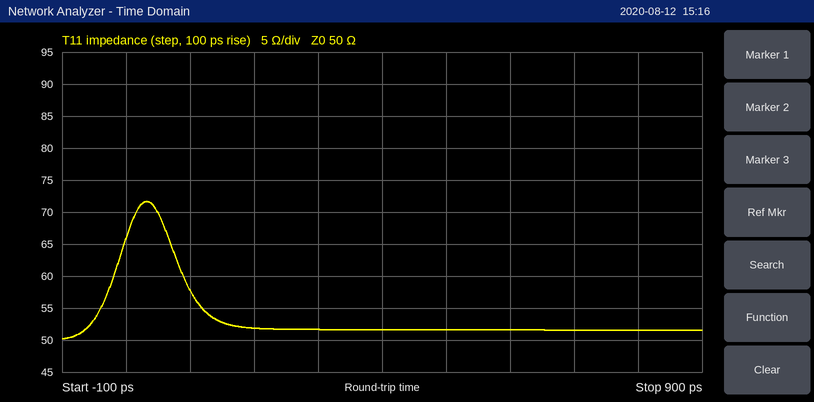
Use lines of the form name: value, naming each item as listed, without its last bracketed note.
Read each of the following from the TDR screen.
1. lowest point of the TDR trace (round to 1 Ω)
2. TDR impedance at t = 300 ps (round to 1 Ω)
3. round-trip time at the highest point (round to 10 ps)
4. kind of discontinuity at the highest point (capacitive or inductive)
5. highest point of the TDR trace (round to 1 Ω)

lowest point of the TDR trace: 50 Ω
TDR impedance at t = 300 ps: 52 Ω
round-trip time at the highest point: 30 ps
kind of discontinuity at the highest point: inductive
highest point of the TDR trace: 72 Ω
